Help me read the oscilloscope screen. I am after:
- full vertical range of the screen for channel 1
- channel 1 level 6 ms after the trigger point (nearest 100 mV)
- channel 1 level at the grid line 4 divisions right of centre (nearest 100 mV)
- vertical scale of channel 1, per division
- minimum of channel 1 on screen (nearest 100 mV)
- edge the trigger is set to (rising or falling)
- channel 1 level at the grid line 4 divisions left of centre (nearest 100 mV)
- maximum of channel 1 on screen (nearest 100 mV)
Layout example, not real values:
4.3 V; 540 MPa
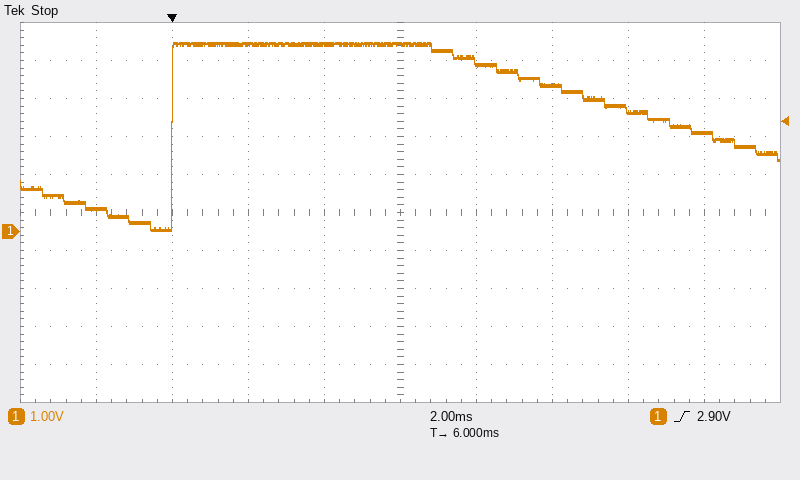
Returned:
10 V; 4.9 V; 2.6 V; 1 V; 0.0 V; rising; 600 mV; 5.0 V
